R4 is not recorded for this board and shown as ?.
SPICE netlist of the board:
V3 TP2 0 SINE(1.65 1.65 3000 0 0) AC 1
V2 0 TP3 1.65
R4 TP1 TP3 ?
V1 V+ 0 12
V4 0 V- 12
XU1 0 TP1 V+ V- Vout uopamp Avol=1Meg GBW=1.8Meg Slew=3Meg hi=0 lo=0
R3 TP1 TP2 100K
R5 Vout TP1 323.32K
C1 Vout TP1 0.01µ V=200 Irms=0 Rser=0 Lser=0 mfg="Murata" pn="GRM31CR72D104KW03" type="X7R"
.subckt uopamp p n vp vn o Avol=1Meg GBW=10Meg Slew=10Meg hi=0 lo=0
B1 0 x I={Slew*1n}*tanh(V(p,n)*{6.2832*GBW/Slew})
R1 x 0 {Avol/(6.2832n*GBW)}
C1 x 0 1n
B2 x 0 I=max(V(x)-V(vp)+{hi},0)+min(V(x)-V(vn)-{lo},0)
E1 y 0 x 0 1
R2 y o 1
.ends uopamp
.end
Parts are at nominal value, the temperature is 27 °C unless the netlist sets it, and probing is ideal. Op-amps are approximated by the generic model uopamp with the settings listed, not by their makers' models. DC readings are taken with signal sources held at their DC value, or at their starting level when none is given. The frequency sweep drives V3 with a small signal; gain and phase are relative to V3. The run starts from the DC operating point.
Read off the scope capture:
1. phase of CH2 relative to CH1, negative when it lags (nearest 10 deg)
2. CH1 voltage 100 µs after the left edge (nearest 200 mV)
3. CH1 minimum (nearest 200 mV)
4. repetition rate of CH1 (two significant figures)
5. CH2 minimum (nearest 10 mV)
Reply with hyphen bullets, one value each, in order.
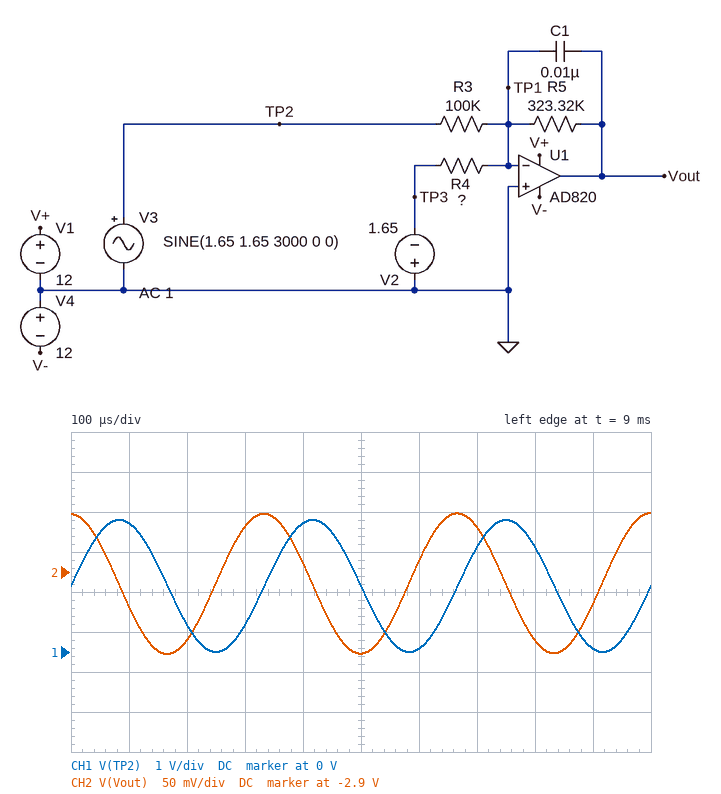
- 90 deg
- 3.2 V
- 0 V
- 3.0 kHz
- -3.00 V
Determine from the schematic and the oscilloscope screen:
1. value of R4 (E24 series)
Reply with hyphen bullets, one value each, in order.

- 220 kΩ
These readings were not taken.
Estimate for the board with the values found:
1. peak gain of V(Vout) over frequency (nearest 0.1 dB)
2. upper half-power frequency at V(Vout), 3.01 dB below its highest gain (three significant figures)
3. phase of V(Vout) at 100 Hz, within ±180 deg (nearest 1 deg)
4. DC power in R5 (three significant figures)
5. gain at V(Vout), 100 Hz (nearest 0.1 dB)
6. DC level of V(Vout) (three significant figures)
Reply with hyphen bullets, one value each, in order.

- 10.2 dB
- 49.2 Hz
- 116 deg
- 26.2 µW
- 3.1 dB
- -2.91 V
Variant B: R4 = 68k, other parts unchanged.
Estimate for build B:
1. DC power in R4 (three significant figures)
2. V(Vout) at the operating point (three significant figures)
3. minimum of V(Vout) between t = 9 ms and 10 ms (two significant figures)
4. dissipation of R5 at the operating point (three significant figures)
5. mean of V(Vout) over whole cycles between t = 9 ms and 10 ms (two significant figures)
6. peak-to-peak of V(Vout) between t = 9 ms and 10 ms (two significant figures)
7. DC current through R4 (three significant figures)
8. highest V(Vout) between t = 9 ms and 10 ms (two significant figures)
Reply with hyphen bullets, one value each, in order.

- 40.0 µW
- 2.51 V
- 2.4 V
- 19.5 µW
- 2.5 V
- 180 mV
- 24.3 µA
- 2.6 V
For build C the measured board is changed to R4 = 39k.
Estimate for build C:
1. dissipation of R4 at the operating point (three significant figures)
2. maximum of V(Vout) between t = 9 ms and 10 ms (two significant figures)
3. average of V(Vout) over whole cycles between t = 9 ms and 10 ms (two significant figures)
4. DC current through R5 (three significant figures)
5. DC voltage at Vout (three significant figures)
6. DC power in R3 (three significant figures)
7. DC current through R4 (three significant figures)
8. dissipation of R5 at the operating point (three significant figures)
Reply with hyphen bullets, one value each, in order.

- 69.8 µW
- 8.4 V
- 8.3 V
- 25.8 µA
- 8.34 V
- 27.2 µW
- 42.3 µA
- 215 µW
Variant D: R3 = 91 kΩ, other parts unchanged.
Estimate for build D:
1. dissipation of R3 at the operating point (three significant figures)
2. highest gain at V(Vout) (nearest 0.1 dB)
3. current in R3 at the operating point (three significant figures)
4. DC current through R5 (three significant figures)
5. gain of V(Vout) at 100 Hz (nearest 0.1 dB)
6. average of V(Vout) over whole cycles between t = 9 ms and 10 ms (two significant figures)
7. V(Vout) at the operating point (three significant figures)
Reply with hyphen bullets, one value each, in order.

- 29.9 µW
- 11.0 dB
- 18.1 µA
- 10.6 µA
- 3.9 dB
- -3.4 V
- -3.44 V
